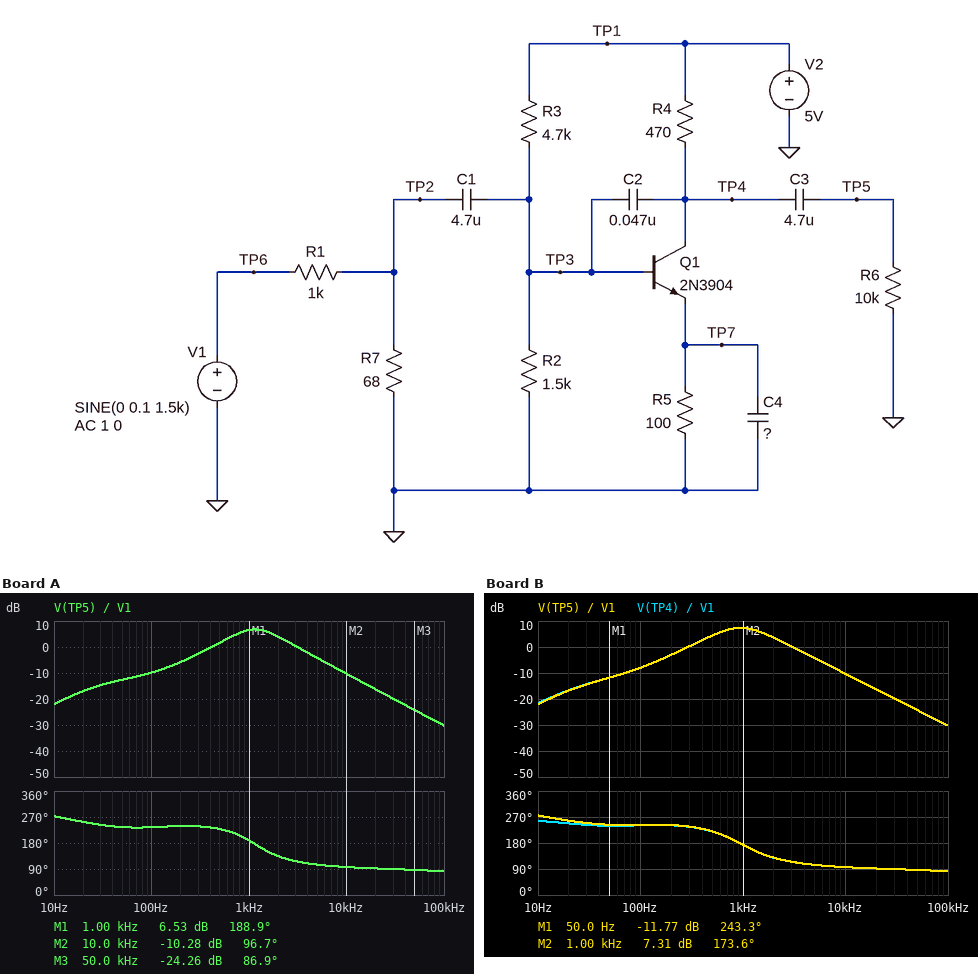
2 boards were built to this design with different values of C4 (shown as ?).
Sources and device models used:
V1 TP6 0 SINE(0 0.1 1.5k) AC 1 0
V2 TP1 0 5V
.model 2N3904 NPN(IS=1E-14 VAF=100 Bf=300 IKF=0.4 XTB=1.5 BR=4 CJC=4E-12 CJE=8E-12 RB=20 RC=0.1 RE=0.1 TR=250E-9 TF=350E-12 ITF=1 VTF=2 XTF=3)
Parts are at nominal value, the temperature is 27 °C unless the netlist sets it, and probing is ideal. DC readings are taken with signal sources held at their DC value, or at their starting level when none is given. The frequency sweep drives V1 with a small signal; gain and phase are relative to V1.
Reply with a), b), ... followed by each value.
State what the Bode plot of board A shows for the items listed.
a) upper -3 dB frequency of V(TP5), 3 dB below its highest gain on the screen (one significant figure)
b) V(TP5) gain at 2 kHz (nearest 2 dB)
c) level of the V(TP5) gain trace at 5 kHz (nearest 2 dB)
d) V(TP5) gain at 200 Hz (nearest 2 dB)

a) 2 kHz
b) 4 dB
c) -4 dB
d) -6 dB
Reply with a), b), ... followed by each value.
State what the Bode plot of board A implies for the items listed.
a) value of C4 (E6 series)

a) 15 µF
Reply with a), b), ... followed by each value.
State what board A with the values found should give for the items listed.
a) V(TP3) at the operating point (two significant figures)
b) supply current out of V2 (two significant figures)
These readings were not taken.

a) 1.2 V
b) 5.7 mA
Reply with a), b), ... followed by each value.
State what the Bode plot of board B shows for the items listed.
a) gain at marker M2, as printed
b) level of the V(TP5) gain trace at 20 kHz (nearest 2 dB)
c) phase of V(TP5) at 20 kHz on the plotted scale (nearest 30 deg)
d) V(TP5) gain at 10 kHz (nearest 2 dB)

a) 7.31 dB
b) -16 dB
c) 90 deg
d) -10 dB
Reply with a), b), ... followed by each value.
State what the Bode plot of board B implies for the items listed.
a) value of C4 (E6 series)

a) 22 µF
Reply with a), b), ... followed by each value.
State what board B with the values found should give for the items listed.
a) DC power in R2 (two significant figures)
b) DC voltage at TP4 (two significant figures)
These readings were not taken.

a) 950 µW
b) 2.7 V
